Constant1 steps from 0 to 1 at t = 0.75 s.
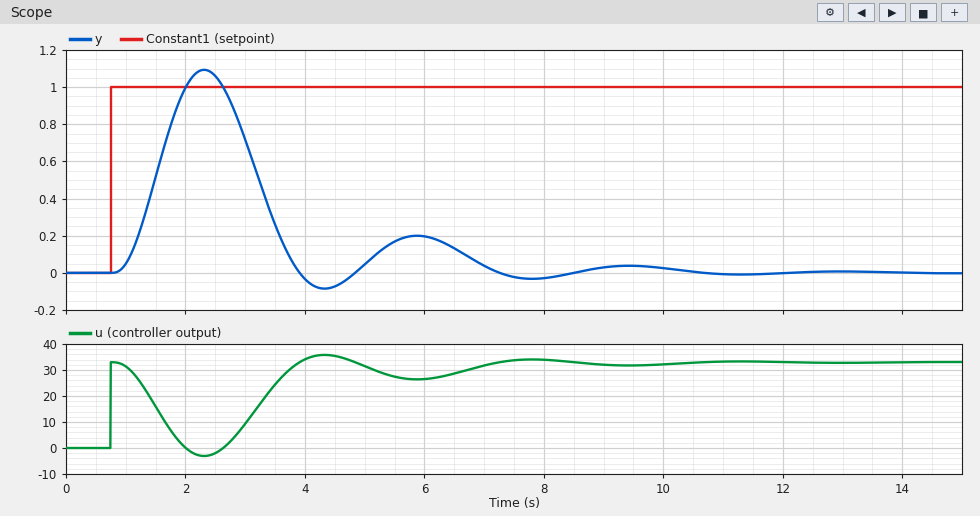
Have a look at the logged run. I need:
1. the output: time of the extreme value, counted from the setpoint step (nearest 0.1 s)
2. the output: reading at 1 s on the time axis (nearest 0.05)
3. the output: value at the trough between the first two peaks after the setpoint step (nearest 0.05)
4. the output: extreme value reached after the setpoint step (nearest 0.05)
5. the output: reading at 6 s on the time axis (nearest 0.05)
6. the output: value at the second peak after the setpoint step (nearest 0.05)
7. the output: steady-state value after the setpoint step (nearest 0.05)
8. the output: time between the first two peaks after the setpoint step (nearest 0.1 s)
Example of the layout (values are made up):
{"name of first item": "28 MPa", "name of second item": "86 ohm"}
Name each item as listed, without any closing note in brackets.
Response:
{"the output: time of the extreme value, counted from the setpoint step": "1.6 s", "the output: reading at 1 s on the time axis": "0.05", "the output: value at the trough between the first two peaks after the setpoint step": "-0.10", "the output: extreme value reached after the setpoint step": "1.10", "the output: reading at 6 s on the time axis": "0.20", "the output: value at the second peak after the setpoint step": "0.20", "the output: steady-state value after the setpoint step": "0.00", "the output: time between the first two peaks after the setpoint step": "3.6 s"}
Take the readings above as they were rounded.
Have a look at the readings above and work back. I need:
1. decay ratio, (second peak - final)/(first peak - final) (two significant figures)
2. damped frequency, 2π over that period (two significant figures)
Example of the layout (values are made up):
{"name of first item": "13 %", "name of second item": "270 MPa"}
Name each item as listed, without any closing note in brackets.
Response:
{"decay ratio, (second peak - final)/(first peak - final)": "0.18", "damped frequency, 2π over that period": "1.7 rad/s"}
